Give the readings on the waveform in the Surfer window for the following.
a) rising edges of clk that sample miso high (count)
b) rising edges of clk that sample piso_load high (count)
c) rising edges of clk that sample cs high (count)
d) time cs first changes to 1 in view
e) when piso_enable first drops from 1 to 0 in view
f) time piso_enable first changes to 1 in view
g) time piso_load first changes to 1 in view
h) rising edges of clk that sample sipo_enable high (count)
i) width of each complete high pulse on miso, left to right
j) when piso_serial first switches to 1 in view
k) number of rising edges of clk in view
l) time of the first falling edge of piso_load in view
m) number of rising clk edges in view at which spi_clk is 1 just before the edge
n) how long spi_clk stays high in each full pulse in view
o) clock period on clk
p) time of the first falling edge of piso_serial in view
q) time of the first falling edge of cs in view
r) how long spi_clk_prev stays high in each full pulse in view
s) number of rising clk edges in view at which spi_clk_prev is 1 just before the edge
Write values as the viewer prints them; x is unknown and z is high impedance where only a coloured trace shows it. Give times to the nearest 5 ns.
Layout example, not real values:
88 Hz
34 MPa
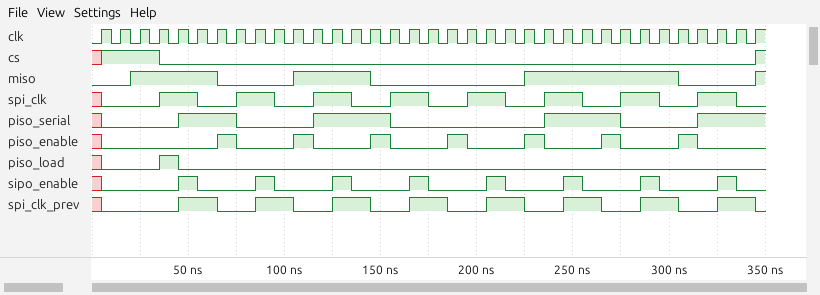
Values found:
17
1
3
5 ns
75 ns
65 ns
35 ns
8
45 ns, 40 ns, 80 ns
45 ns
35
45 ns
16
20 ns, 20 ns, 20 ns, 20 ns, 20 ns, 20 ns, 20 ns, 20 ns
10 ns
75 ns
35 ns
20 ns, 20 ns, 20 ns, 20 ns, 20 ns, 20 ns, 20 ns, 20 ns
16
